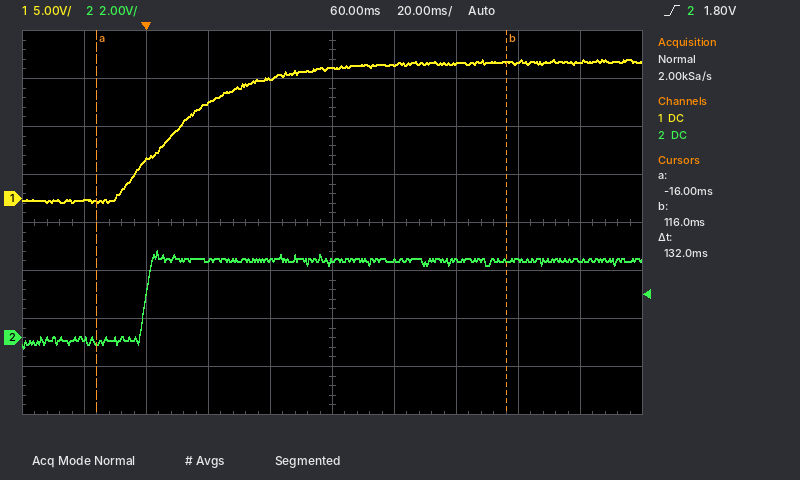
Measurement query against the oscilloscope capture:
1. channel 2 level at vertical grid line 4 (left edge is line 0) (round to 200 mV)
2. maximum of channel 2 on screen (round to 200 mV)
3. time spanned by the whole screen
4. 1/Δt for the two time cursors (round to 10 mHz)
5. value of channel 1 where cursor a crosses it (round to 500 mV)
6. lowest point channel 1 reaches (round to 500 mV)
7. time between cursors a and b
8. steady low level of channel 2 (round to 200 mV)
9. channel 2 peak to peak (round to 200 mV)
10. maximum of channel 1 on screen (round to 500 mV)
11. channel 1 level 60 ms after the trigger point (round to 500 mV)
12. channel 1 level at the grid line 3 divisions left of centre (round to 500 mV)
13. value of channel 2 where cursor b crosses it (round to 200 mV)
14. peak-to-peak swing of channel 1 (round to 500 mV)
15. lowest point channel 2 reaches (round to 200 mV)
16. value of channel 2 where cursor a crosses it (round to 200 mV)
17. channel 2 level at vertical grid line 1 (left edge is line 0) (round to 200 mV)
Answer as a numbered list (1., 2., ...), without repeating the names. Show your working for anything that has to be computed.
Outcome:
1. 3.2 V
2. 3.6 V
3. 200 ms
4. 1 / 132 ms ≈ 7.58 Hz
5. -500 mV
6. -500 mV
7. 132 ms
8. -200 mV
9. 3.6 V − (-400 mV) = 4.0 V
10. 14.5 V
11. 13.5 V
12. 4.0 V
13. 3.2 V
14. 14.5 V − (-500 mV) = 15.0 V
15. -400 mV
16. -200 mV
17. 0.0 V
